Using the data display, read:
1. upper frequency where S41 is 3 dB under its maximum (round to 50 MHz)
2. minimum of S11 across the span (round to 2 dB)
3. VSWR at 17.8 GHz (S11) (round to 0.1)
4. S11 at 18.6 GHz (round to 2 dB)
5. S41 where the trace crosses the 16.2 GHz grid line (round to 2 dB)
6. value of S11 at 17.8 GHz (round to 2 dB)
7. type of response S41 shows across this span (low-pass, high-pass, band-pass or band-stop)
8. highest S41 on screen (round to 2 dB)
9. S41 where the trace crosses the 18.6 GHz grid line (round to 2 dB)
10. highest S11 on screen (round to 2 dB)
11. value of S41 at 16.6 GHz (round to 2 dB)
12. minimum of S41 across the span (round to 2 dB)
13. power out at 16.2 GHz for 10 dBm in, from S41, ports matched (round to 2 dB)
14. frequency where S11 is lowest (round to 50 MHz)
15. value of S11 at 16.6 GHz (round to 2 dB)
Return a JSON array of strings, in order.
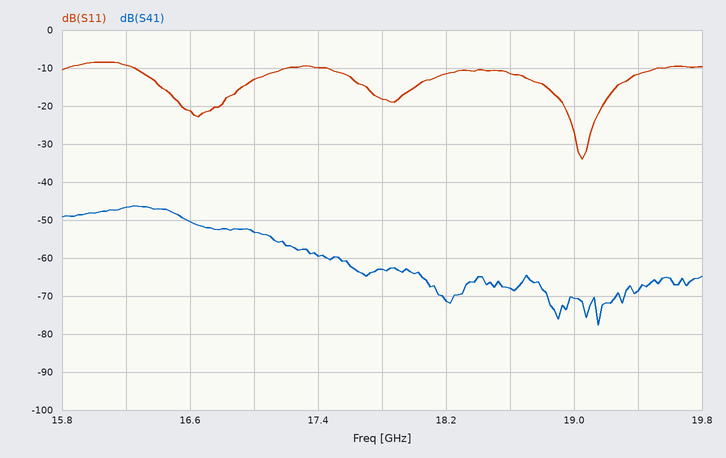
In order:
["16.55 GHz", "-34 dB", "1.3", "-12 dB", "-46 dB", "-18 dB", "low-pass", "-46 dB", "-68 dB", "-8 dB", "-50 dB", "-78 dB", "-36 dBm", "19.05 GHz", "-22 dB"]
